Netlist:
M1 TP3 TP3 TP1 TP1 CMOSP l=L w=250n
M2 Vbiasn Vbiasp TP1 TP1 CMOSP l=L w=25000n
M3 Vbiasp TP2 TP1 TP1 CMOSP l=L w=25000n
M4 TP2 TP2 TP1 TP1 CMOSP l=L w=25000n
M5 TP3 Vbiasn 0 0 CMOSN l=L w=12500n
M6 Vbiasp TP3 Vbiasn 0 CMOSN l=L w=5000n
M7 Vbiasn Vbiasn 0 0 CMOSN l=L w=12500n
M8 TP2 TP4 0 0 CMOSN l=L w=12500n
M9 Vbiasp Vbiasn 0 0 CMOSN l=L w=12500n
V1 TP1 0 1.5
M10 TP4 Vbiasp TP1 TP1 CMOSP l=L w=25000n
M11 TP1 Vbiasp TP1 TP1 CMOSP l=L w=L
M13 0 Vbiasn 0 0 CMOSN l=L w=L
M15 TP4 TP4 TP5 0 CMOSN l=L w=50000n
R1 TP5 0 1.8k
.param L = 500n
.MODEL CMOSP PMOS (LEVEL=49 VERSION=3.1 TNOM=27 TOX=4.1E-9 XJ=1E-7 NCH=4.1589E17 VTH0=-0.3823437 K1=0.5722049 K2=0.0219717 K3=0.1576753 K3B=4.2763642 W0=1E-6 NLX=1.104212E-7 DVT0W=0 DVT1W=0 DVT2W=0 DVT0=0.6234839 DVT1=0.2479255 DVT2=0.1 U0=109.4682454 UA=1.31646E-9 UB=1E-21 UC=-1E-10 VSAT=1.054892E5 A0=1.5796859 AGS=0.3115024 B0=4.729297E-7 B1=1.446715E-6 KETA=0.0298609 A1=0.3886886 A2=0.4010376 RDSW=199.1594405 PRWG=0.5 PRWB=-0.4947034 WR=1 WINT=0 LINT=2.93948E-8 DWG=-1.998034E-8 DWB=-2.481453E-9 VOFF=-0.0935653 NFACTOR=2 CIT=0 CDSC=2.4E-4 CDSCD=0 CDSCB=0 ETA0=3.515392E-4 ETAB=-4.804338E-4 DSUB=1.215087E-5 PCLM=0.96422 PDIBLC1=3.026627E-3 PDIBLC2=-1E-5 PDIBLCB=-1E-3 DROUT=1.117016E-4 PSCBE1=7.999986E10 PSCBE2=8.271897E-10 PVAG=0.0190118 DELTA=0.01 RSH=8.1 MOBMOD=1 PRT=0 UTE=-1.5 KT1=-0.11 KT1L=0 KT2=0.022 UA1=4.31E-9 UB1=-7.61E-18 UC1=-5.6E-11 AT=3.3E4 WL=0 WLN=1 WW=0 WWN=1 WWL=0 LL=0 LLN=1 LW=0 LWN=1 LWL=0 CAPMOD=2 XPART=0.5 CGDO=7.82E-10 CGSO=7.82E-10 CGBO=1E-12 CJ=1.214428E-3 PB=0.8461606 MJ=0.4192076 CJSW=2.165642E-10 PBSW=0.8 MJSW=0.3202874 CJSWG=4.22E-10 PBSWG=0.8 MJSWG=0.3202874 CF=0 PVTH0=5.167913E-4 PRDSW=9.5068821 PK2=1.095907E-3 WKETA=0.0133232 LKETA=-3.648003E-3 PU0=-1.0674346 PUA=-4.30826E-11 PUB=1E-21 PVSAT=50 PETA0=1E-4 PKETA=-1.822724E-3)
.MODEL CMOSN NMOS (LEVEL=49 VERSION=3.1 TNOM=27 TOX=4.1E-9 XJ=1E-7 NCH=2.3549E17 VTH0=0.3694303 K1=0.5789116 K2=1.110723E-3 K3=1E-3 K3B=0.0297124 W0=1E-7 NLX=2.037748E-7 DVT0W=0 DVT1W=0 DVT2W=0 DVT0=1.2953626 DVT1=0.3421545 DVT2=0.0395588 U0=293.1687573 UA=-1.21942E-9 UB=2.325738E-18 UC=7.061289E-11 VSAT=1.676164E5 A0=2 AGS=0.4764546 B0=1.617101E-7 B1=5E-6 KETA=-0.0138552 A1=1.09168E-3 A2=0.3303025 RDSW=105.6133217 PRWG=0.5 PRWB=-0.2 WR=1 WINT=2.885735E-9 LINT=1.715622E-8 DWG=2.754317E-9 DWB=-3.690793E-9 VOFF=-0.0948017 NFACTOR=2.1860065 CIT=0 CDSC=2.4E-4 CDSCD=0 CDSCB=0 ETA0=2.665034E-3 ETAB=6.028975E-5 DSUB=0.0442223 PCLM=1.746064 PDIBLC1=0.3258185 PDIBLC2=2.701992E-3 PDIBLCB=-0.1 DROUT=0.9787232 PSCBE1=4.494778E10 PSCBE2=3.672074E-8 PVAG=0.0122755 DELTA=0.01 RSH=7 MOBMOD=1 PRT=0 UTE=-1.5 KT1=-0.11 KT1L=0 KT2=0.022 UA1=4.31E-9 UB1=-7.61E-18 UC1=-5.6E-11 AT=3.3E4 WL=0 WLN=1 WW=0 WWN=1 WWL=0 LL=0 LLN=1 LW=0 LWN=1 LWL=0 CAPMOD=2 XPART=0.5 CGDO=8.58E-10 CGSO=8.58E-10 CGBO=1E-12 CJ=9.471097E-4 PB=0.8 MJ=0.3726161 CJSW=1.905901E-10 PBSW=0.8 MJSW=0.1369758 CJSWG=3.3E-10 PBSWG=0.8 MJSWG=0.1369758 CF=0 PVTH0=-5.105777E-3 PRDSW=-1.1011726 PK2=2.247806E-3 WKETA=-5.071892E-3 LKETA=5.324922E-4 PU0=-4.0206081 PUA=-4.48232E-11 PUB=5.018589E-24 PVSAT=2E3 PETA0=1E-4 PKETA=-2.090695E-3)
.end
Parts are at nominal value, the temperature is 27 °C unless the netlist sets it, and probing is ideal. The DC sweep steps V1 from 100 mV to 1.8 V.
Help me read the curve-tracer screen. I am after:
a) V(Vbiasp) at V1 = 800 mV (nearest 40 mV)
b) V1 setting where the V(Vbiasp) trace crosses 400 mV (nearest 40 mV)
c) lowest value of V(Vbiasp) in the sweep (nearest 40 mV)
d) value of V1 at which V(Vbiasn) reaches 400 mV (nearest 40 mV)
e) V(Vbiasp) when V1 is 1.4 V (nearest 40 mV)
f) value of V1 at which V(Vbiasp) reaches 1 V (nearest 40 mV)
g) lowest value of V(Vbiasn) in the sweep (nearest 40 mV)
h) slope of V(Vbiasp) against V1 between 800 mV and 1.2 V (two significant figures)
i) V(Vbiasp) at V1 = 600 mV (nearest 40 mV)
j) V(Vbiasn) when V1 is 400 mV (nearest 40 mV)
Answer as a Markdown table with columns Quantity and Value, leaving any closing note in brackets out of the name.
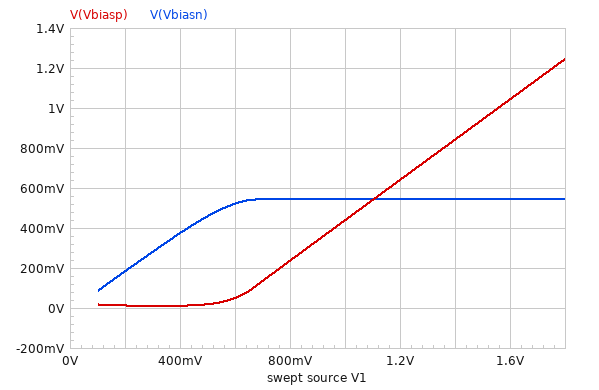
| Quantity | Value |
|---|---|
| V(Vbiasp) at V1 = 800 mV | 240 mV |
| V1 setting where the V(Vbiasp) trace crosses 400 mV | 960 mV |
| lowest value of V(Vbiasp) in the sweep | 0 V |
| value of V1 at which V(Vbiasn) reaches 400 mV | 440 mV |
| V(Vbiasp) when V1 is 1.4 V | 840 mV |
| value of V1 at which V(Vbiasp) reaches 1 V | 1.56 V |
| lowest value of V(Vbiasn) in the sweep | 80 mV |
| slope of V(Vbiasp) against V1 between 800 mV and 1.2 V | 1.0 V/V |
| V(Vbiasp) at V1 = 600 mV | 40 mV |
| V(Vbiasn) when V1 is 400 mV | 360 mV |
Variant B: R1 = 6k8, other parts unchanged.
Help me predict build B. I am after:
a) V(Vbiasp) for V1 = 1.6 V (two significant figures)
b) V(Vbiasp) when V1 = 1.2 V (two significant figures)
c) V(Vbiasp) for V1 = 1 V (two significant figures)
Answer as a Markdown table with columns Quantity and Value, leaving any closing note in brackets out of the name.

| Quantity | Value |
|---|---|
| V(Vbiasp) for V1 = 1.6 V | 1.1 V |
| V(Vbiasp) when V1 = 1.2 V | 730 mV |
| V(Vbiasp) for V1 = 1 V | 530 mV |
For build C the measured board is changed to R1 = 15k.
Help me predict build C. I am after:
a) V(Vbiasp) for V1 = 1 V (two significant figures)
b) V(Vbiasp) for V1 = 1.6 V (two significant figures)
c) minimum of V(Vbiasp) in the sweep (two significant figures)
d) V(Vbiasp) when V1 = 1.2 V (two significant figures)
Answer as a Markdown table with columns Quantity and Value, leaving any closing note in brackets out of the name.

| Quantity | Value |
|---|---|
| V(Vbiasp) for V1 = 1 V | 570 mV |
| V(Vbiasp) for V1 = 1.6 V | 1.2 V |
| minimum of V(Vbiasp) in the sweep | 12 mV |
| V(Vbiasp) when V1 = 1.2 V | 770 mV |
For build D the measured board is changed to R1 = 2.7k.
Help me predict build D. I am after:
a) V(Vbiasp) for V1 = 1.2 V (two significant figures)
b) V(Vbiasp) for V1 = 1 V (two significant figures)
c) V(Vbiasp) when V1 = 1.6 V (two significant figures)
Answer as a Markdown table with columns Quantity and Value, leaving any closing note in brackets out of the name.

| Quantity | Value |
|---|---|
| V(Vbiasp) for V1 = 1.2 V | 670 mV |
| V(Vbiasp) for V1 = 1 V | 470 mV |
| V(Vbiasp) when V1 = 1.6 V | 1.1 V |
